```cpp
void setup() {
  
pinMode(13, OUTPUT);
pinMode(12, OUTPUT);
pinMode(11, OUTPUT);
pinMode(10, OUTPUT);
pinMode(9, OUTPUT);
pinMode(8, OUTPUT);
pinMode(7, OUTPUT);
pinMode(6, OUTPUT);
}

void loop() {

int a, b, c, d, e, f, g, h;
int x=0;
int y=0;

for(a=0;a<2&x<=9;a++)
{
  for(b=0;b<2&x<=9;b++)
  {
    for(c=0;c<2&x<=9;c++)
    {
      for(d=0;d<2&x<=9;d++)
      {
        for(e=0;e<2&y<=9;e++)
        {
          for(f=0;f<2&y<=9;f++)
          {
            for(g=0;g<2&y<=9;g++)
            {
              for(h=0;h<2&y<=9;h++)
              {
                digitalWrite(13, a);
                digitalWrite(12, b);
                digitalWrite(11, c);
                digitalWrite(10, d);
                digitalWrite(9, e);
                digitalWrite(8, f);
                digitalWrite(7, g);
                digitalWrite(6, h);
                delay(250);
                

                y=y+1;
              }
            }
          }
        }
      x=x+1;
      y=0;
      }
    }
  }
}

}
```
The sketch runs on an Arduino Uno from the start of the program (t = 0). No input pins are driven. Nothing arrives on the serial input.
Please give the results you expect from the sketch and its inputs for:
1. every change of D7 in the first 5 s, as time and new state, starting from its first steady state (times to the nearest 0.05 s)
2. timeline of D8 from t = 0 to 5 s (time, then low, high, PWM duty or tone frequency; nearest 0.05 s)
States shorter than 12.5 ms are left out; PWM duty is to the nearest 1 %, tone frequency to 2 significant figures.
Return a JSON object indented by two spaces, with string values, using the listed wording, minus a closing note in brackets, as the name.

{
  "every change of D7 in the first 5 s, as time and new state, starting from its first steady state": "0 s low; 0.5 s high; 1 s low; 1.5 s high; 2 s low; 3 s high; 3.5 s low; 4 s high; 4.5 s low",
  "timeline of D8 from t = 0 to 5 s": "0 s low; 1 s high; 2 s low; 3.5 s high; 4.5 s low"
}
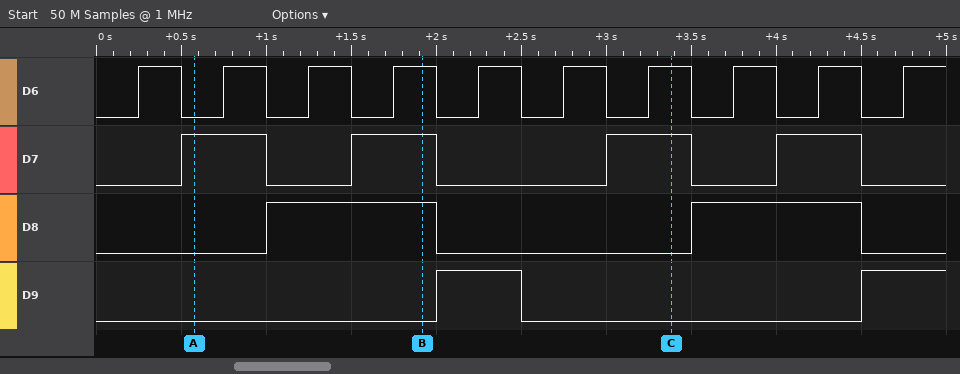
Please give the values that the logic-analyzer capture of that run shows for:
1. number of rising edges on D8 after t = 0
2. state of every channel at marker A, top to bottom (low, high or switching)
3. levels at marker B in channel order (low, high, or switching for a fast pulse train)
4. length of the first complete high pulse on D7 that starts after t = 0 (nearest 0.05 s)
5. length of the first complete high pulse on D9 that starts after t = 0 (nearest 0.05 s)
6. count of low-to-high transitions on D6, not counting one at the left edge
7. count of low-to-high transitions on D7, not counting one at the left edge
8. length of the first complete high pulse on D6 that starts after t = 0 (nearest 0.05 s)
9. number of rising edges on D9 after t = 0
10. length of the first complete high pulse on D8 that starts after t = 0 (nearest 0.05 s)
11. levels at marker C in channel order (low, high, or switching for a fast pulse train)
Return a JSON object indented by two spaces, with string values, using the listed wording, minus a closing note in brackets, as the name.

{
  "number of rising edges on D8 after t = 0": "2",
  "state of every channel at marker A, top to bottom": "D6 low, D7 high, D8 low, D9 low",
  "levels at marker B in channel order": "D6 high, D7 high, D8 high, D9 low",
  "length of the first complete high pulse on D7 that starts after t = 0": "0.50 s",
  "length of the first complete high pulse on D9 that starts after t = 0": "0.50 s",
  "count of low-to-high transitions on D6, not counting one at the left edge": "10",
  "count of low-to-high transitions on D7, not counting one at the left edge": "4",
  "length of the first complete high pulse on D6 that starts after t = 0": "0.25 s",
  "number of rising edges on D9 after t = 0": "2",
  "length of the first complete high pulse on D8 that starts after t = 0": "1.00 s",
  "levels at marker C in channel order": "D6 high, D7 high, D8 low, D9 low"
}
